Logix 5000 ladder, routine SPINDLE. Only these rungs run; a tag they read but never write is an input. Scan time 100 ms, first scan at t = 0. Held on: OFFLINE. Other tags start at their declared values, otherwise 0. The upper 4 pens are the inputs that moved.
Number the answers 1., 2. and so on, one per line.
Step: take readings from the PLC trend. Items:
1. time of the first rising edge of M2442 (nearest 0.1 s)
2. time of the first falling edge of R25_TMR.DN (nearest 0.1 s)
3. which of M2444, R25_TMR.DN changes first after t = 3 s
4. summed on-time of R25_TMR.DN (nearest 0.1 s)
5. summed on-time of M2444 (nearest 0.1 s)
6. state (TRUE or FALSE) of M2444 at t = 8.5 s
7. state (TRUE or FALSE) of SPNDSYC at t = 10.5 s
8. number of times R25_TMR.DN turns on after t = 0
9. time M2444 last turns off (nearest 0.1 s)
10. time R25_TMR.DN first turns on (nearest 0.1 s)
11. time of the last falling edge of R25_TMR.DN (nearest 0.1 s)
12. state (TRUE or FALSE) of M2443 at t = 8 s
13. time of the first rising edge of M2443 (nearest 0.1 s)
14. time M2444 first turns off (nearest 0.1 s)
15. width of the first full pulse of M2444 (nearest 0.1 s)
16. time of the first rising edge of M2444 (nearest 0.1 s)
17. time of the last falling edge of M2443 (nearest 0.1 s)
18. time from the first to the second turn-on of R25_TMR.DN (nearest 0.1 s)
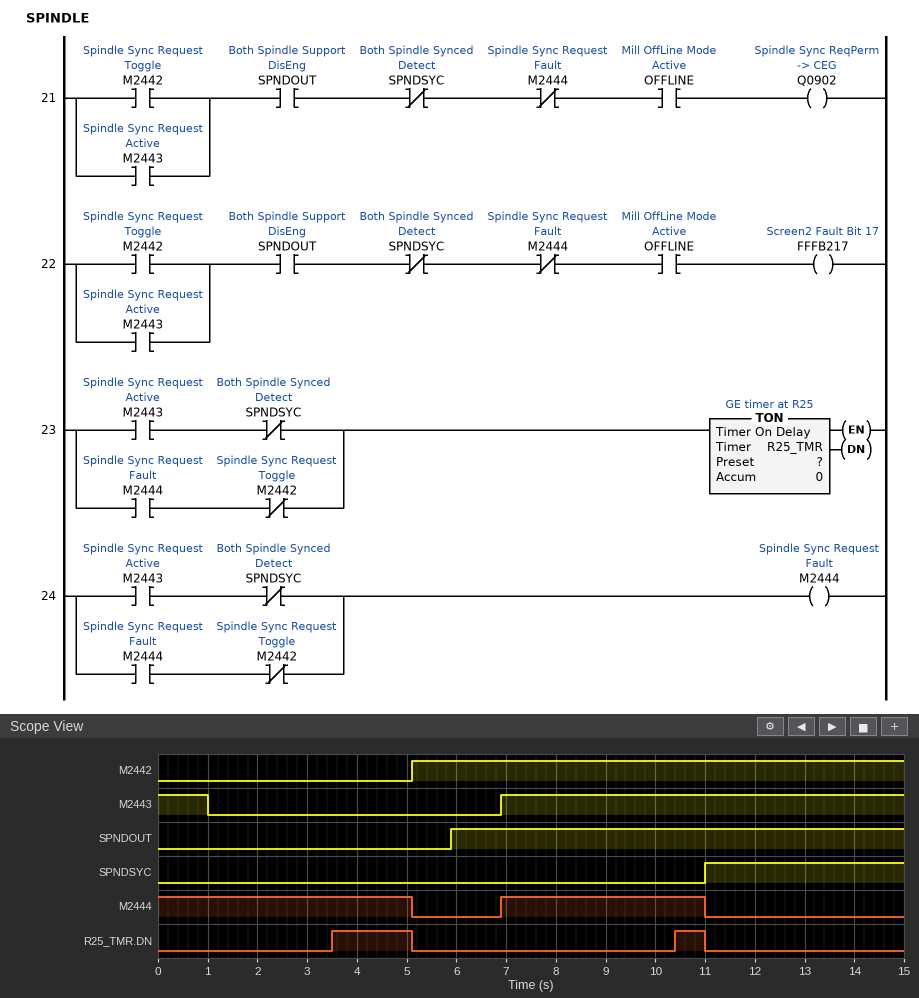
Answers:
1. 5.1 s
2. 5.1 s
3. R25_TMR.DN
4. 2.2 s
5. 9.2 s
6. TRUE
7. FALSE
8. 2
9. 11.0 s
10. 3.5 s
11. 11.0 s
12. TRUE
13. 6.9 s
14. 5.1 s
15. 4.1 s
16. 6.9 s
17. 1.0 s
18. 6.9 s
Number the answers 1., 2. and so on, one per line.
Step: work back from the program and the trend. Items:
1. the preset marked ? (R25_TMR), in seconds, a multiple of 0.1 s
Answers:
1. 3.5 s
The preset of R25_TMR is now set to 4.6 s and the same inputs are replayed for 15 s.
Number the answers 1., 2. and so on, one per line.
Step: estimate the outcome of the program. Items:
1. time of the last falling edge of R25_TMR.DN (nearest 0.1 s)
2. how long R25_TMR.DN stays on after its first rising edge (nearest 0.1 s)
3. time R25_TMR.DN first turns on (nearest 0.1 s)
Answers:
1. 5.1 s
2. 0.5 s
3. 4.6 s
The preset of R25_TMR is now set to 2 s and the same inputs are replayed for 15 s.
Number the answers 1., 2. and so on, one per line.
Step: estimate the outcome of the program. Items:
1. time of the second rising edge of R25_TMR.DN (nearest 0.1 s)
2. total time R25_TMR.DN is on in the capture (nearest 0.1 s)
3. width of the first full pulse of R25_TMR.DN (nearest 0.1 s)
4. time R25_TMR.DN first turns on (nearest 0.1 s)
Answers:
1. 8.9 s
2. 5.2 s
3. 3.1 s
4. 2.0 s
